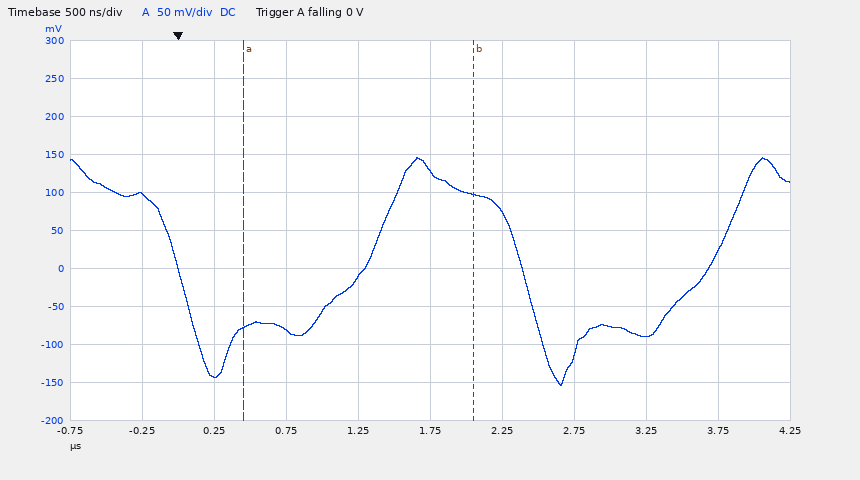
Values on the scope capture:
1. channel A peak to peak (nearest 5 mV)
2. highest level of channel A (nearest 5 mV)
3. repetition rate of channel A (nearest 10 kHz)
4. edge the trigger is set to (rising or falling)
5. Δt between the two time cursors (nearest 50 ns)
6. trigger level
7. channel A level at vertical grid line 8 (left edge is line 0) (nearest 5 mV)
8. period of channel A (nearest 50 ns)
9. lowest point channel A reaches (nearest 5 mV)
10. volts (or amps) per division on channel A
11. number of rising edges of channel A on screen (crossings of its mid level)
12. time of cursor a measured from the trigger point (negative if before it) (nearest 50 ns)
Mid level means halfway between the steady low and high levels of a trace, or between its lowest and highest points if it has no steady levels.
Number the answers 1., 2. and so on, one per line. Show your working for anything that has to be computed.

1. 145 mV − (-155 mV) = 300 mV
2. 145 mV
3. 1 / 2.40 µs ≈ 417 kHz, so 420 kHz to the nearest 10 kHz
4. falling
5. 1.60 µs
6. 0 V
7. -90 mV
8. 2.40 µs
9. -155 mV
10. 50 mV
11. 2
12. +450 ns
